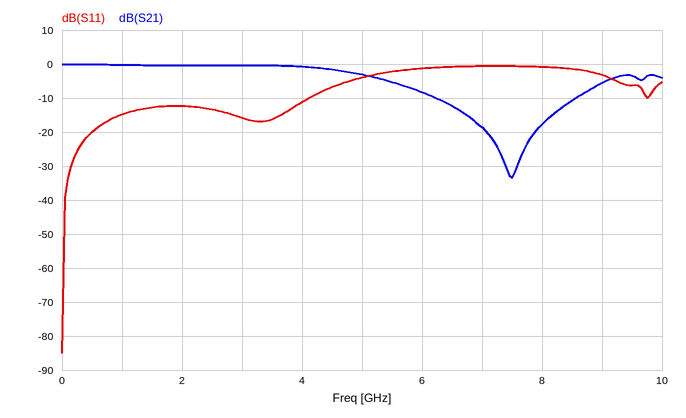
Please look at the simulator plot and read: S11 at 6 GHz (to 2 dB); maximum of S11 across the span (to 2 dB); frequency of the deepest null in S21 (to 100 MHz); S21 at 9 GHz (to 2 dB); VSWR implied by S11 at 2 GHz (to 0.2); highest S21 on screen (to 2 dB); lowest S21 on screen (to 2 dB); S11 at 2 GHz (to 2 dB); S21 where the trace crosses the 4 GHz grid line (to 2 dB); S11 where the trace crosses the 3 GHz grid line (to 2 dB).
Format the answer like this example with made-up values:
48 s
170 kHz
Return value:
-2 dB
0 dB
7.5 GHz
-6 dB
1.6
0 dB
-34 dB
-12 dB
0 dB
-16 dB
